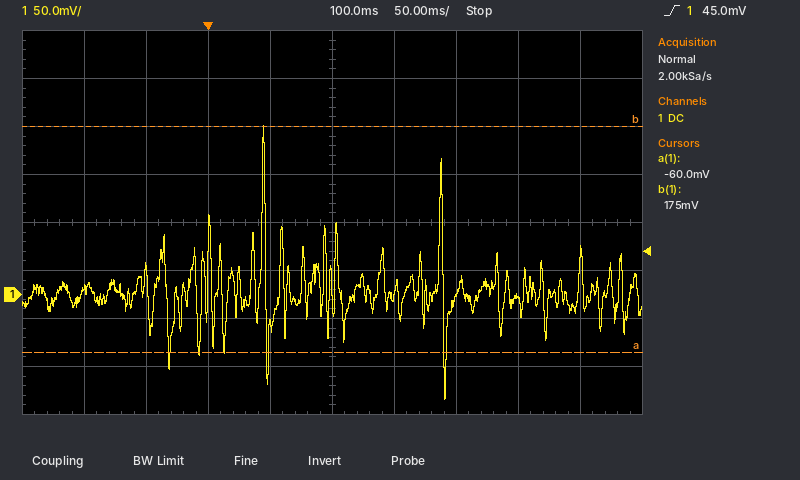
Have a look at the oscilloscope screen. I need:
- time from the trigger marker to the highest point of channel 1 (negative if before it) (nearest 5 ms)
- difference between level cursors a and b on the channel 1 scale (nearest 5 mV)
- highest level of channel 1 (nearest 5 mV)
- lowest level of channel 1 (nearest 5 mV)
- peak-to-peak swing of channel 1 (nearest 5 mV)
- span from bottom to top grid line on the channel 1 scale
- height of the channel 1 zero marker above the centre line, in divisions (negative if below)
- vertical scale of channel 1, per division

+45 ms
235 mV
175 mV
-110 mV
285 mV
400 mV
-1.5 div
50 mV
